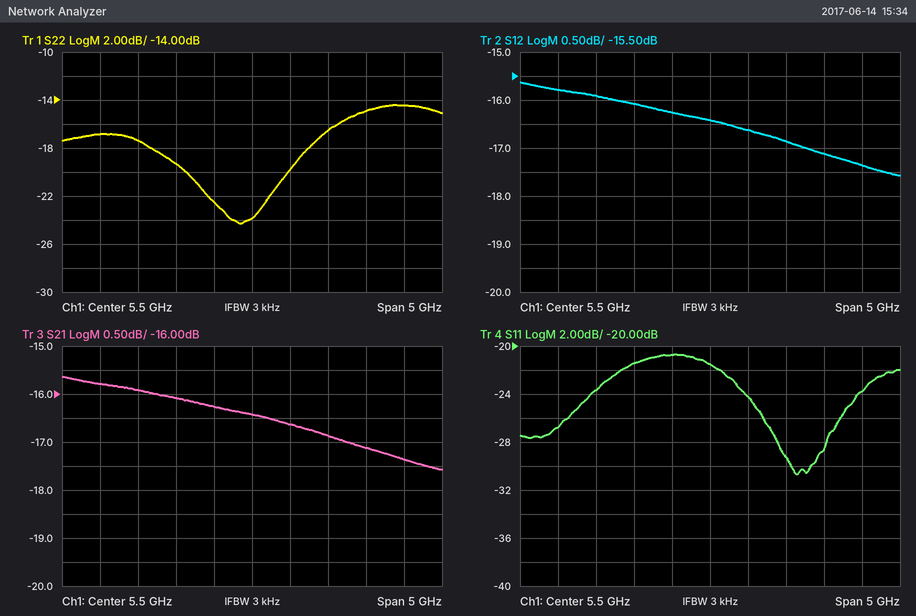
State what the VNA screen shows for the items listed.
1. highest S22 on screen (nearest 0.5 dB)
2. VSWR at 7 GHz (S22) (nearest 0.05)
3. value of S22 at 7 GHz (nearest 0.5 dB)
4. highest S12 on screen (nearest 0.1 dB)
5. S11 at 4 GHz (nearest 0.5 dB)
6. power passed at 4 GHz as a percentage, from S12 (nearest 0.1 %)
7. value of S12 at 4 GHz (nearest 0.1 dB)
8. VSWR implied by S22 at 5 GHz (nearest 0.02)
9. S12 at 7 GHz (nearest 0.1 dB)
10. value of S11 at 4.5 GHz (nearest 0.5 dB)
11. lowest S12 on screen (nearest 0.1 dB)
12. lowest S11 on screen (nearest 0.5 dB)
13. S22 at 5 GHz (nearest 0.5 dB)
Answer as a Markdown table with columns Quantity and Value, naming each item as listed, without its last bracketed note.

| Quantity | Value |
|---|---|
| highest S22 on screen | -14.5 dB |
| VSWR at 7 GHz (S22) | 1.45 |
| value of S22 at 7 GHz | -15.0 dB |
| highest S12 on screen | -15.6 dB |
| S11 at 4 GHz | -23.5 dB |
| power passed at 4 GHz as a percentage, from S12 | 2.6 % |
| value of S12 at 4 GHz | -15.9 dB |
| VSWR implied by S22 at 5 GHz | 1.16 |
| S12 at 7 GHz | -17.1 dB |
| value of S11 at 4.5 GHz | -21.5 dB |
| lowest S12 on screen | -17.6 dB |
| lowest S11 on screen | -30.5 dB |
| S22 at 5 GHz | -22.5 dB |
